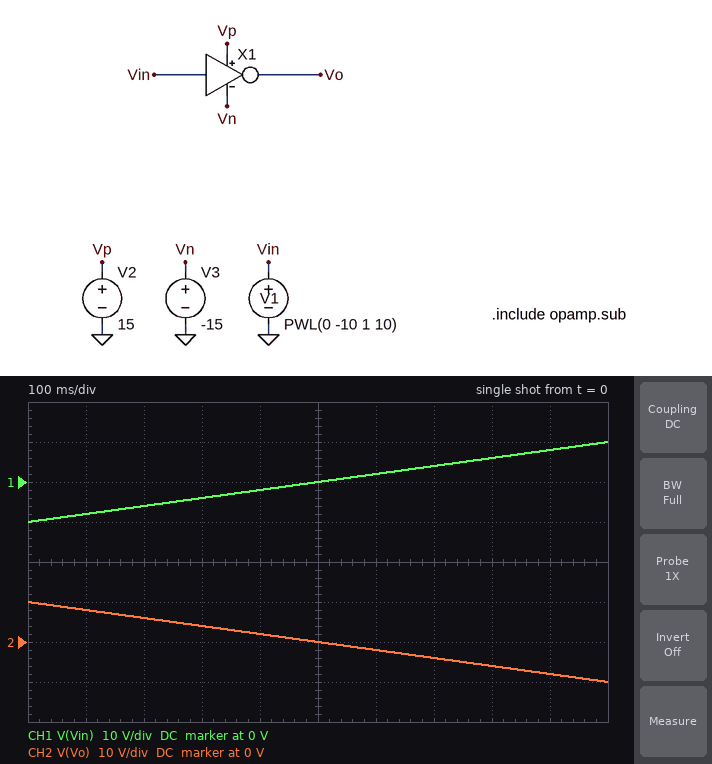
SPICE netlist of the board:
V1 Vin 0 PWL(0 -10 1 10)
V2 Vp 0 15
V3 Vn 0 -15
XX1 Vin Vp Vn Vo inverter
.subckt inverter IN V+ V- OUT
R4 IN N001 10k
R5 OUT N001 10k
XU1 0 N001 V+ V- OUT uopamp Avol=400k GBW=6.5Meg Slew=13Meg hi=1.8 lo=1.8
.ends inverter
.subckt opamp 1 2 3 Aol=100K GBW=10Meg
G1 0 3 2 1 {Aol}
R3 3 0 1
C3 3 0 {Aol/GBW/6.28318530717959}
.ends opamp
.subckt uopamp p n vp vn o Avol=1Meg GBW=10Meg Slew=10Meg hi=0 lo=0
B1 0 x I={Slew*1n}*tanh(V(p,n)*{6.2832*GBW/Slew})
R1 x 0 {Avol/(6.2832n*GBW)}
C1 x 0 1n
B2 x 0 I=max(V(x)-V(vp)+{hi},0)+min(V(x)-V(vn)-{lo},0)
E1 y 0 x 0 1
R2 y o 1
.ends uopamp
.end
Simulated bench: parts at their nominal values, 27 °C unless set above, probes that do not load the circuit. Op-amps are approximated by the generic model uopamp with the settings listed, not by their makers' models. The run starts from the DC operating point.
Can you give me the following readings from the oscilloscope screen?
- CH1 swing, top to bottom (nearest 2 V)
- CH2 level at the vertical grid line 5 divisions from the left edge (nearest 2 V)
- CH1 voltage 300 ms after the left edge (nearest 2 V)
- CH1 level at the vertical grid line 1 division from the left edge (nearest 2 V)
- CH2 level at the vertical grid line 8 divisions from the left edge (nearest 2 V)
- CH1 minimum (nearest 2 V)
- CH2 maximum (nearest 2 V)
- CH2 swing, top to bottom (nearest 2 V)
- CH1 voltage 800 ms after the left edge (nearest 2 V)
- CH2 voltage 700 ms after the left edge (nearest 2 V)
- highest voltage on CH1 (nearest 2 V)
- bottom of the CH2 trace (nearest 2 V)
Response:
20 V
0 V
-4 V
-8 V
-6 V
-10 V
10 V
20 V
6 V
-4 V
10 V
-10 V
